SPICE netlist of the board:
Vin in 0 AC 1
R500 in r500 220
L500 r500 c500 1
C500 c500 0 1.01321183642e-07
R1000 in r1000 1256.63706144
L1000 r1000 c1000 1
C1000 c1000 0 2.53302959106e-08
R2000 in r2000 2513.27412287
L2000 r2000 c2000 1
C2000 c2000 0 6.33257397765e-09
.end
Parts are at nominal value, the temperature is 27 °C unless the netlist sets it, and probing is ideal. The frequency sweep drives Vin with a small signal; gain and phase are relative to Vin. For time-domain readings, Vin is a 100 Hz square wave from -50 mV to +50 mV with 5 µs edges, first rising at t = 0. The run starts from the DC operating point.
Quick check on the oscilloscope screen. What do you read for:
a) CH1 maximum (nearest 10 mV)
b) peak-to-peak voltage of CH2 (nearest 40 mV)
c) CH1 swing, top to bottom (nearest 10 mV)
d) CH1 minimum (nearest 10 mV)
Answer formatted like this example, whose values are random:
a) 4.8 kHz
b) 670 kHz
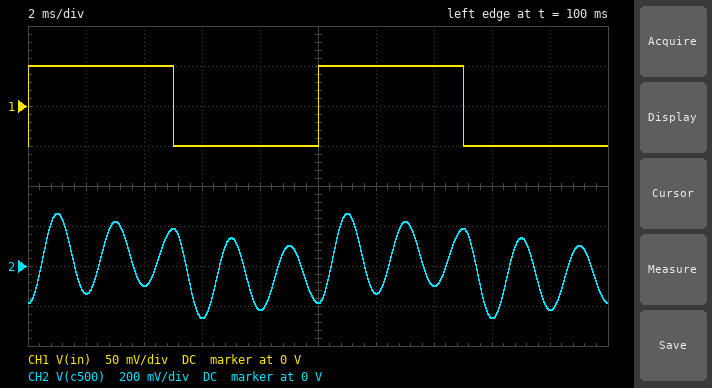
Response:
a) 50 mV
b) 520 mV
c) 100 mV
d) -50 mV
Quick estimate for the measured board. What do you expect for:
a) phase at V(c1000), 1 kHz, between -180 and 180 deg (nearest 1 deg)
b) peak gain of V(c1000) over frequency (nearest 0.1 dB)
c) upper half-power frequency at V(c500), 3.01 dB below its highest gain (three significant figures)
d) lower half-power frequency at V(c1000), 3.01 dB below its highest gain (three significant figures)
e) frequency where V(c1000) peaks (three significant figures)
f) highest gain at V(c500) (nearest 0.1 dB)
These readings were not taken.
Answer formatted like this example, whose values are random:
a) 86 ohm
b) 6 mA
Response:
a) -90 deg
b) 14.0 dB
c) 517 Hz
d) 884 Hz
e) 990 Hz
f) 23.1 dB
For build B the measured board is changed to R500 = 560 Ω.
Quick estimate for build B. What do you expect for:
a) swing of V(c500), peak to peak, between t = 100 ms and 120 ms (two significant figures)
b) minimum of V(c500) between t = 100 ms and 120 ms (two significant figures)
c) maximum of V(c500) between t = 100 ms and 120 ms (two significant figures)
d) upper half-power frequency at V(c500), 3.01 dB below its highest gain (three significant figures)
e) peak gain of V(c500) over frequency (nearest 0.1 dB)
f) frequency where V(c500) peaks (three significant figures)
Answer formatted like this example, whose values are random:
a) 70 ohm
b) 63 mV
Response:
a) 300 mV
b) -150 mV
c) 150 mV
d) 539 Hz
e) 15.0 dB
f) 496 Hz
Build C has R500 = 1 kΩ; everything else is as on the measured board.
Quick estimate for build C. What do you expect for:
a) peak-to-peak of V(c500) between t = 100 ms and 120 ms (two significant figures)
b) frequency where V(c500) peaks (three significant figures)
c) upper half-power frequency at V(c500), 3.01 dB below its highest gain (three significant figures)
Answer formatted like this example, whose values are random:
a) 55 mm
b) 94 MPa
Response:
a) 230 mV
b) 487 Hz
c) 562 Hz
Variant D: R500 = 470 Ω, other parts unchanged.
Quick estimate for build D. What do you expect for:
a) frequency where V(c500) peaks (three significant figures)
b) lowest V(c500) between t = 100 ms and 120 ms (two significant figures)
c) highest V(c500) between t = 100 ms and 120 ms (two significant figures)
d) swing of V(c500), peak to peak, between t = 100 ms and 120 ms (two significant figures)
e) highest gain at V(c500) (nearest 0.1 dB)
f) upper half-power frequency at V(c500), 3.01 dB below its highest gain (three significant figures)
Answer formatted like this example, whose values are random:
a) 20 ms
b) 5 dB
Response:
a) 497 Hz
b) -160 mV
c) 160 mV
d) 330 mV
e) 16.5 dB
f) 533 Hz
